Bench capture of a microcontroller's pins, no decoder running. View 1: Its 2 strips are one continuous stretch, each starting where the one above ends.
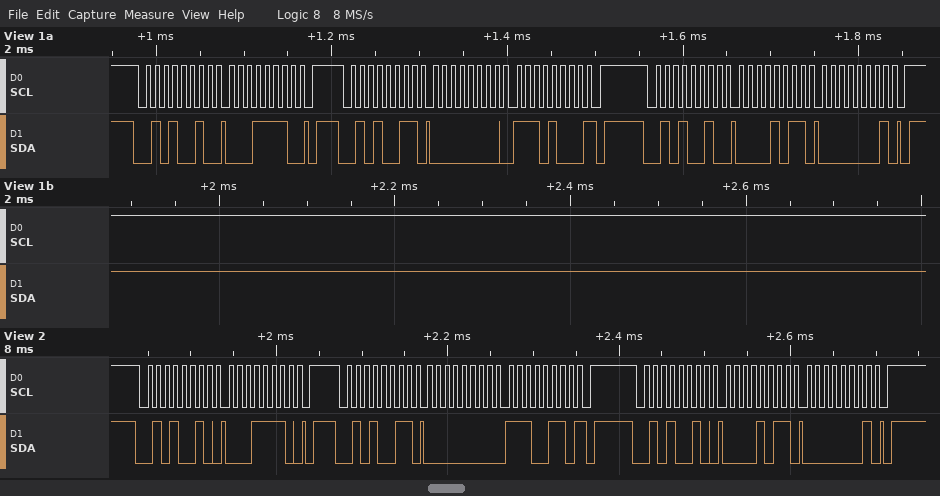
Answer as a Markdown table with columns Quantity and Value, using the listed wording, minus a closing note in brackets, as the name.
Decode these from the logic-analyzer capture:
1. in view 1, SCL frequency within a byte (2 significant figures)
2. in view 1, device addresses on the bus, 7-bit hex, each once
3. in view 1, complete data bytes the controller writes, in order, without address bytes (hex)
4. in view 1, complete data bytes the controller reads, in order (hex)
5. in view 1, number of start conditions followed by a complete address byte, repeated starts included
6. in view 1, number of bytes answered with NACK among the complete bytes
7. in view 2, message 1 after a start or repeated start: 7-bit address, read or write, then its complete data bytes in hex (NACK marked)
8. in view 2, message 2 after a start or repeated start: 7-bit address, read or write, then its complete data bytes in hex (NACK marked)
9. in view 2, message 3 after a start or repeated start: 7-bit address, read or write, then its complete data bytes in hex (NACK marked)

| Quantity | Value |
|---|---|
| in view 1, SCL frequency within a byte | 100 kHz |
| in view 1, device addresses on the bus, 7-bit hex, each once | 0x29 |
| in view 1, complete data bytes the controller writes, in order, without address bytes | 1E 0B 01 |
| in view 1, complete data bytes the controller reads, in order | 00 E8 |
| in view 1, number of start conditions followed by a complete address byte, repeated starts included | 3 |
| in view 1, number of bytes answered with NACK among the complete bytes | 1 |
| in view 2, message 1 after a start or repeated start: 7-bit address, read or write, then its complete data bytes in hex | 0x29 write: 1E |
| in view 2, message 2 after a start or repeated start: 7-bit address, read or write, then its complete data bytes in hex | 0x29 read: 00 E6 NACK |
| in view 2, message 3 after a start or repeated start: 7-bit address, read or write, then its complete data bytes in hex | 0x29 write: 0B 01 |
